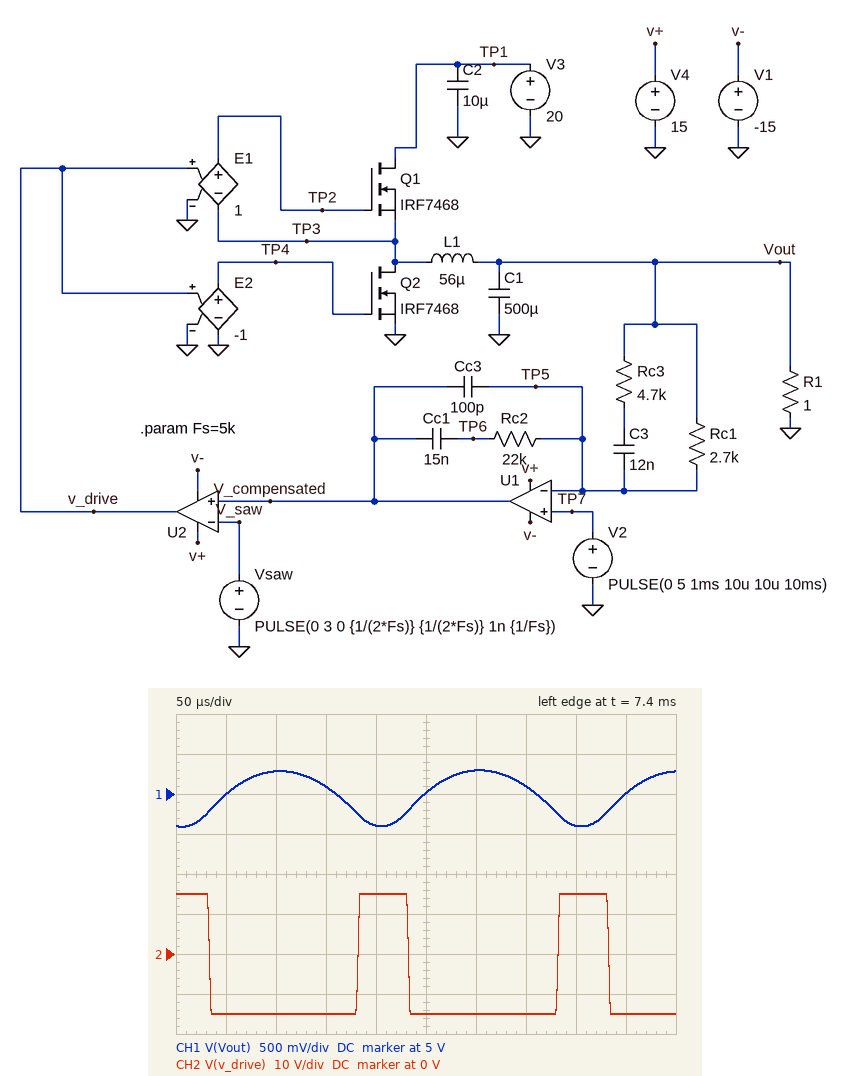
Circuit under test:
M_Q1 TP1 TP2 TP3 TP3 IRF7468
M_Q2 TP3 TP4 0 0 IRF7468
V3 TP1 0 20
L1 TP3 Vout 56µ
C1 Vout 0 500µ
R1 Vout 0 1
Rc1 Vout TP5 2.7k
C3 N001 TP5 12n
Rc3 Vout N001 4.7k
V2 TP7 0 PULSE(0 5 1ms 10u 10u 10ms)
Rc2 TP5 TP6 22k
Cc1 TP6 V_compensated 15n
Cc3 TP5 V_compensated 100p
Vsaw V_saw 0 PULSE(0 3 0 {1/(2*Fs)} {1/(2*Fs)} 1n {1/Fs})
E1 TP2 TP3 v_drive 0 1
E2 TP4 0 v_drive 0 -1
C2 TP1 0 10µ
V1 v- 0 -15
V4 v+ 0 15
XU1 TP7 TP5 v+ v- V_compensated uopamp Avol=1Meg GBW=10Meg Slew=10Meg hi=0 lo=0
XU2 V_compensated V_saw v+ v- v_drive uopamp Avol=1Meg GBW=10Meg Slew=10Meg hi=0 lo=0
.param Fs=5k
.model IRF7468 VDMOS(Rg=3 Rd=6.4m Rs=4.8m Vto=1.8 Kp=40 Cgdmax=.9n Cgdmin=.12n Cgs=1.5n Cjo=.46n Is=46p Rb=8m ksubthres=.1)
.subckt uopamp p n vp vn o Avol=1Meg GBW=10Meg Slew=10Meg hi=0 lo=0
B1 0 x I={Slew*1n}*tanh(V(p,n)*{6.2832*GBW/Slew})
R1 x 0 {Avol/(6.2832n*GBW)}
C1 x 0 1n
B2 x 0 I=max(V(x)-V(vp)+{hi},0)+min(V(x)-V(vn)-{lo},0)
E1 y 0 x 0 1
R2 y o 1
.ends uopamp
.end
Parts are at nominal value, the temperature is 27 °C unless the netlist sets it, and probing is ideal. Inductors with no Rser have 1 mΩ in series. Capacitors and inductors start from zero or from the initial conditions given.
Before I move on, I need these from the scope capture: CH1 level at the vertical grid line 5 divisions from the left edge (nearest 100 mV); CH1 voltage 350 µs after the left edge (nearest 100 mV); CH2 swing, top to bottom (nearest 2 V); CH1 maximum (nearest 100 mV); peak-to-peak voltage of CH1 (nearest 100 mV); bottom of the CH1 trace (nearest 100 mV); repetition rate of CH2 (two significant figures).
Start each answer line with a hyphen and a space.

- 5.0 V
- 5.1 V
- 30 V
- 5.3 V
- 700 mV
- 4.6 V
- 5.0 kHz
